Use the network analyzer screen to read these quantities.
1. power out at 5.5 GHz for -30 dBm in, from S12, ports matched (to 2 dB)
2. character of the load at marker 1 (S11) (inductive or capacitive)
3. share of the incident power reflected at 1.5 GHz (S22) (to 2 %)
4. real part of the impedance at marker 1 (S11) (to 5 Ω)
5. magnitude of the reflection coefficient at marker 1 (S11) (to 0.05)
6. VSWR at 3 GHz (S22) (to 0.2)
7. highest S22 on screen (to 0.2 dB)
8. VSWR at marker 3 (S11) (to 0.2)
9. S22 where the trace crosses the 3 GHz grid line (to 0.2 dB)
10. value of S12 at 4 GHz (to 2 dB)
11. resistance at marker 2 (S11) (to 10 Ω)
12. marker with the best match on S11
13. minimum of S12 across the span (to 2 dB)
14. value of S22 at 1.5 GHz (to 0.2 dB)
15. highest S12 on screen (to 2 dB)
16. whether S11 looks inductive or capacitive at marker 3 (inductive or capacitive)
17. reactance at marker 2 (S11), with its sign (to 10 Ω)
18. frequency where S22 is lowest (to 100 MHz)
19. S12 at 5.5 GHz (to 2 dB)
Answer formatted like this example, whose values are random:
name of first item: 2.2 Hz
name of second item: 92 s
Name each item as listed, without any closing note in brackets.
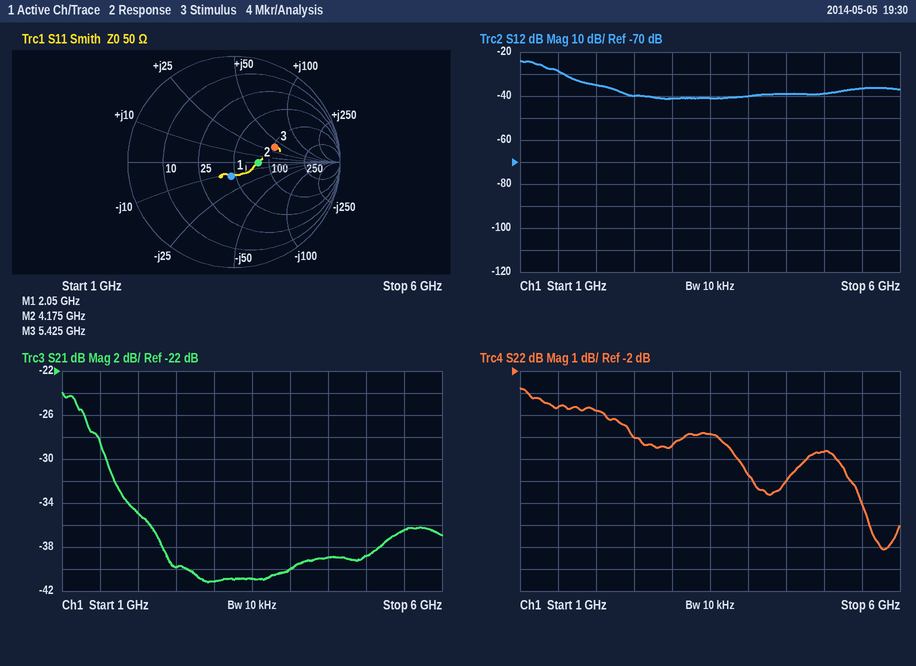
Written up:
power out at 5.5 GHz for -30 dBm in, from S12, ports matched: -66 dBm
character of the load at marker 1 (S11): capacitive
share of the incident power reflected at 1.5 GHz (S22): 44 %
real part of the impedance at marker 1 (S11): 45 Ω
magnitude of the reflection coefficient at marker 1 (S11): 0.15
VSWR at 3 GHz (S22): 3.4
highest S22 on screen: -2.8 dB
VSWR at marker 3 (S11): 2.4
S22 where the trace crosses the 3 GHz grid line: -5.4 dB
value of S12 at 4 GHz: -40 dB
resistance at marker 2 (S11): 80 Ω
marker with the best match on S11: marker 1
minimum of S12 across the span: -42 dB
value of S22 at 1.5 GHz: -3.6 dB
highest S12 on screen: -24 dB
whether S11 looks inductive or capacitive at marker 3: inductive
reactance at marker 2 (S11), with its sign: 0 Ω
frequency where S22 is lowest: 5.8 GHz
S12 at 5.5 GHz: -36 dB
